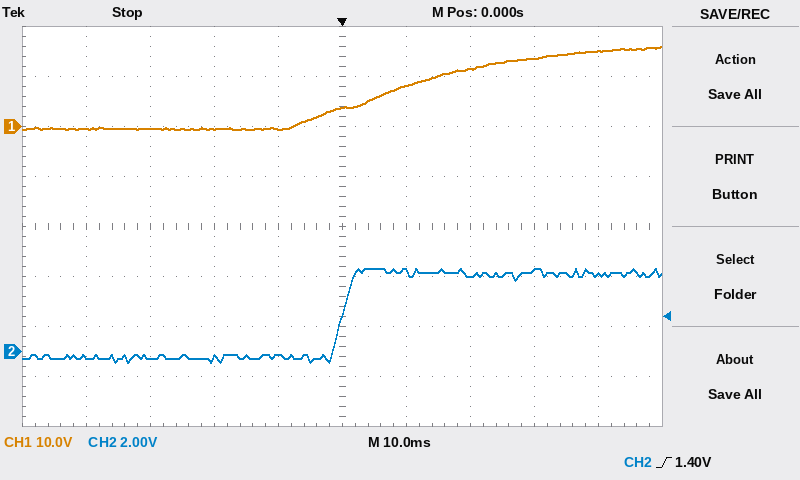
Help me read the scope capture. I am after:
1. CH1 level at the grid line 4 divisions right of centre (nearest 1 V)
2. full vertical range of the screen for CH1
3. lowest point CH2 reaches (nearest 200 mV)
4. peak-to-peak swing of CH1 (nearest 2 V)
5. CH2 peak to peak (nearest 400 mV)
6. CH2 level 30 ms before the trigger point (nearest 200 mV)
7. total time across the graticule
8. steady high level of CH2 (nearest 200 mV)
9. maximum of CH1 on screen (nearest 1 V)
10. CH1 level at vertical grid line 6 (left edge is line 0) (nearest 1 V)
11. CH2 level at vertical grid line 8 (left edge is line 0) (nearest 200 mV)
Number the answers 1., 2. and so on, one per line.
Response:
1. 15 V
2. 80 V
3. -400 mV
4. 16 V
5. 3.6 V
6. -200 mV
7. 100 ms
8. 3.2 V
9. 16 V
10. 8 V
11. 3.2 V
